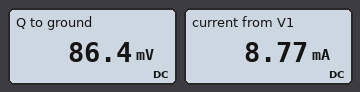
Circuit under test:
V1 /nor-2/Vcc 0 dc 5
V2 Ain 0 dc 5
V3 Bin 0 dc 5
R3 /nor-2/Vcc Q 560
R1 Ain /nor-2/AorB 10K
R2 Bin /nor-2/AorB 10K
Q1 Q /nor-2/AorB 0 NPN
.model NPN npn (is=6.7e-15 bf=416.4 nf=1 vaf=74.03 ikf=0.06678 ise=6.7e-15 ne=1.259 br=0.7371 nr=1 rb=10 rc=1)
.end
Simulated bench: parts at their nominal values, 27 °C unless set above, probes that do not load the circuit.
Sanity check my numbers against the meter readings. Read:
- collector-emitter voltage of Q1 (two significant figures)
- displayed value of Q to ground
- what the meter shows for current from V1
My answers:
86 mV
86.4 mV
8.77 mA
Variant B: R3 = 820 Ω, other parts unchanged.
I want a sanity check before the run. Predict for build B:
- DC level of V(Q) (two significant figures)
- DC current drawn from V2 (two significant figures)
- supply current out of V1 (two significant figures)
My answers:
74 mV
430 µA
6.0 mA
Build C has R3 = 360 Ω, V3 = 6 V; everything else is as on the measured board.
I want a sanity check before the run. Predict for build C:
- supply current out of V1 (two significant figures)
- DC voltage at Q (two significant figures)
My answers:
14 mA
100 mV
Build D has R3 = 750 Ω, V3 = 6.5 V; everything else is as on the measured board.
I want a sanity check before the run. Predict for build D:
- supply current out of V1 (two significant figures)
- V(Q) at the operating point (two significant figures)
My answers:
6.6 mA
73 mV
